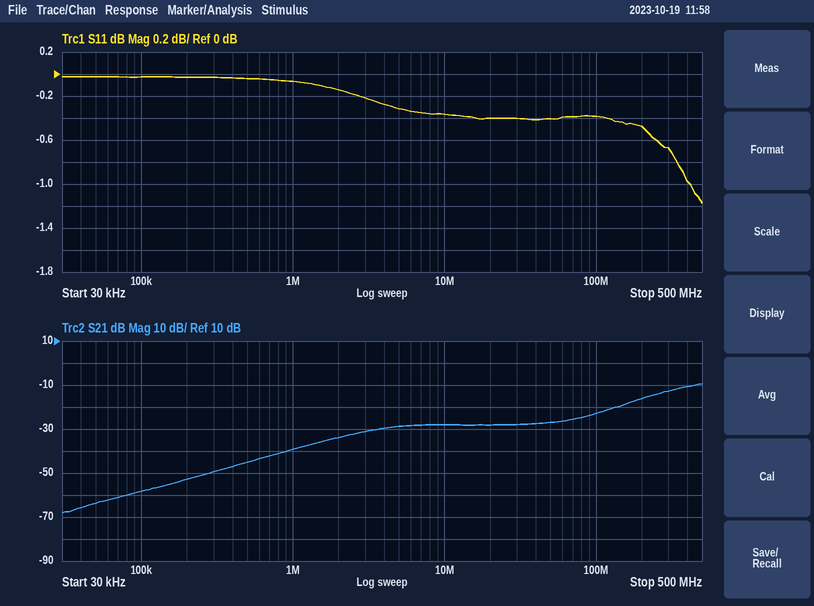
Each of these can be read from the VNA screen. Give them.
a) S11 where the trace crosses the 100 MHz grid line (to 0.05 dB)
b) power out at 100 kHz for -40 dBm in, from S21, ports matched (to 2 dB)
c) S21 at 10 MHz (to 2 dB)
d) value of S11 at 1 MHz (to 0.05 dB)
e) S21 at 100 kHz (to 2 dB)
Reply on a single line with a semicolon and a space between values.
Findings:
-0.40 dB; -98 dBm; -28 dB; -0.05 dB; -58 dB
